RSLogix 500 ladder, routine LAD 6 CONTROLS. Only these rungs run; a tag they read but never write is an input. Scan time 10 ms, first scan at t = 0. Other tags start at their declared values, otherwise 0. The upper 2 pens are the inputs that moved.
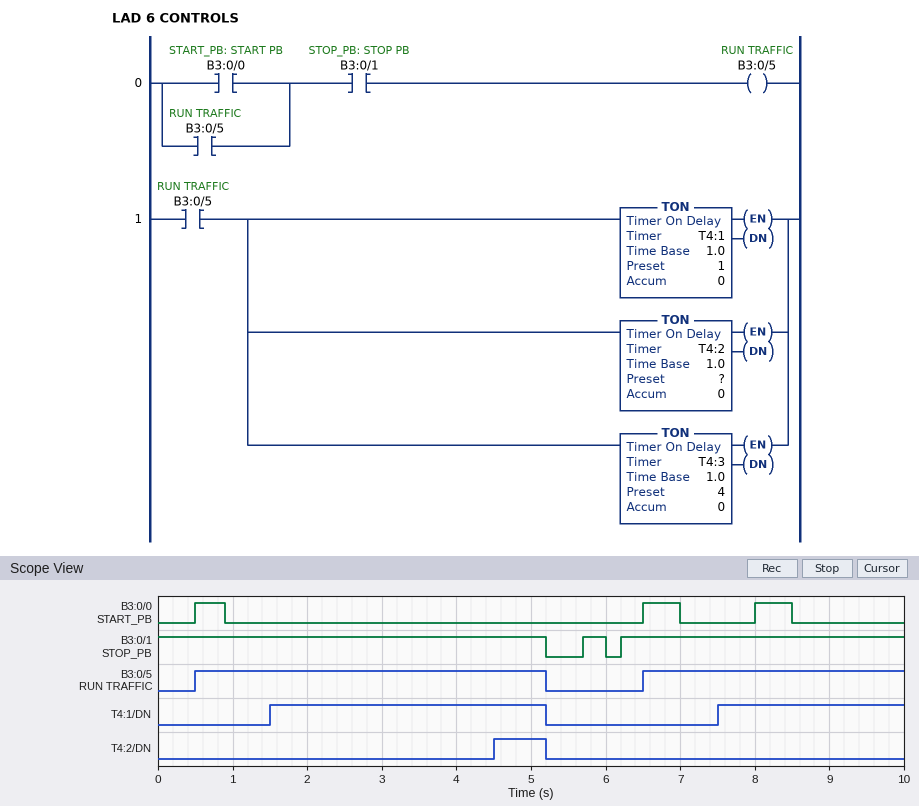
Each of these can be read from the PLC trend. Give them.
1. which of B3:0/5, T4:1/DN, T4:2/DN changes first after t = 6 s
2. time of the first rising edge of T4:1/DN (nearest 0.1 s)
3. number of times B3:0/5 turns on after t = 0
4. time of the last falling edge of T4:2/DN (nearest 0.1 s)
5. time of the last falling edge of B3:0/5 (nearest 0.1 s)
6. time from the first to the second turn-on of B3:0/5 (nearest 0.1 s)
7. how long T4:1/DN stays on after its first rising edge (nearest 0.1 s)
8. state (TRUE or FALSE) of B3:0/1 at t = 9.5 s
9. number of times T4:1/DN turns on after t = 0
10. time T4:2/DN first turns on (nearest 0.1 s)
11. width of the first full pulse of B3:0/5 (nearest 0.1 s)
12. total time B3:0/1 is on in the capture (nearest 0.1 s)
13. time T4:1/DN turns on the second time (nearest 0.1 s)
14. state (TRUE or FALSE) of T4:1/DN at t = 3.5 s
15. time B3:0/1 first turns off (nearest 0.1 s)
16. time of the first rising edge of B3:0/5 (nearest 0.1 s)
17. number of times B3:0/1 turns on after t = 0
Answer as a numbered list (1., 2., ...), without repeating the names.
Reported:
1. B3:0/5
2. 1.5 s
3. 2
4. 5.2 s
5. 5.2 s
6. 6.0 s
7. 3.7 s
8. TRUE
9. 2
10. 4.5 s
11. 4.7 s
12. 9.3 s
13. 7.5 s
14. TRUE
15. 5.2 s
16. 0.5 s
17. 2
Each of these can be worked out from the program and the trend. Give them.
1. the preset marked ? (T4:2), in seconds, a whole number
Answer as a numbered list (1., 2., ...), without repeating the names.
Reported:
1. 4 s
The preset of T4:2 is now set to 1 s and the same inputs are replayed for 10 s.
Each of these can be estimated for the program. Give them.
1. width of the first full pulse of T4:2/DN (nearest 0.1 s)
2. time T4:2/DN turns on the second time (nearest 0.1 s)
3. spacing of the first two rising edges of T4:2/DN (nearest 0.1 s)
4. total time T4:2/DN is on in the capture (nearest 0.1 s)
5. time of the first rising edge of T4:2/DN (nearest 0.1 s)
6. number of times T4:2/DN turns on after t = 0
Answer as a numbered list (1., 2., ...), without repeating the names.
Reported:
1. 3.7 s
2. 7.5 s
3. 6.0 s
4. 6.2 s
5. 1.5 s
6. 2
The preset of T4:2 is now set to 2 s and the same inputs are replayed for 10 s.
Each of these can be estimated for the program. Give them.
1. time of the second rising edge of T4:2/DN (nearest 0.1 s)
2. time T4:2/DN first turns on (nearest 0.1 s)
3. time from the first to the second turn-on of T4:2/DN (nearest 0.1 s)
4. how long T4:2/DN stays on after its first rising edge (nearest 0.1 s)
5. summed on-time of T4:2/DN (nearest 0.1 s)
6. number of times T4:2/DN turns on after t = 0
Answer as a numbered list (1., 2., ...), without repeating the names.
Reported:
1. 8.5 s
2. 2.5 s
3. 6.0 s
4. 2.7 s
5. 4.2 s
6. 2
